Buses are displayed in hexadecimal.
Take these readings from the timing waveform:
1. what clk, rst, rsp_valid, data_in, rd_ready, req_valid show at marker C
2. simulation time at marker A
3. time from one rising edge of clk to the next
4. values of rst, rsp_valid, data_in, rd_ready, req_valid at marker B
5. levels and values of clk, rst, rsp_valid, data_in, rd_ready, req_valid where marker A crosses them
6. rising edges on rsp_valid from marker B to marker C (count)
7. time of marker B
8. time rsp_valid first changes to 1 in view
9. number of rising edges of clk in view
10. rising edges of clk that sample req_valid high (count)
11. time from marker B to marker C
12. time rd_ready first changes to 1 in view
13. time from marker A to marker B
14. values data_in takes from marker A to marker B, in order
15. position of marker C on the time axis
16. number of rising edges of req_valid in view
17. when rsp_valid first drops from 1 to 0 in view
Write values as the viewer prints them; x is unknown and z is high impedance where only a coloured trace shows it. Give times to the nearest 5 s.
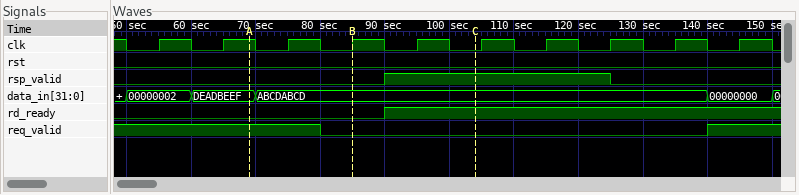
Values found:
clk=0, rst=0, rsp_valid=1, data_in=ABCDABCD, rd_ready=1, req_valid=0
70 s
10 s
rst=0, rsp_valid=0, data_in=ABCDABCD, rd_ready=0, req_valid=0
clk=1, rst=0, rsp_valid=0, data_in=DEADBEEF, rd_ready=0, req_valid=1
1
85 s
90 s
10
4
20 s
90 s
15 s
DEADBEEF, ABCDABCD
105 s
1
125 s
